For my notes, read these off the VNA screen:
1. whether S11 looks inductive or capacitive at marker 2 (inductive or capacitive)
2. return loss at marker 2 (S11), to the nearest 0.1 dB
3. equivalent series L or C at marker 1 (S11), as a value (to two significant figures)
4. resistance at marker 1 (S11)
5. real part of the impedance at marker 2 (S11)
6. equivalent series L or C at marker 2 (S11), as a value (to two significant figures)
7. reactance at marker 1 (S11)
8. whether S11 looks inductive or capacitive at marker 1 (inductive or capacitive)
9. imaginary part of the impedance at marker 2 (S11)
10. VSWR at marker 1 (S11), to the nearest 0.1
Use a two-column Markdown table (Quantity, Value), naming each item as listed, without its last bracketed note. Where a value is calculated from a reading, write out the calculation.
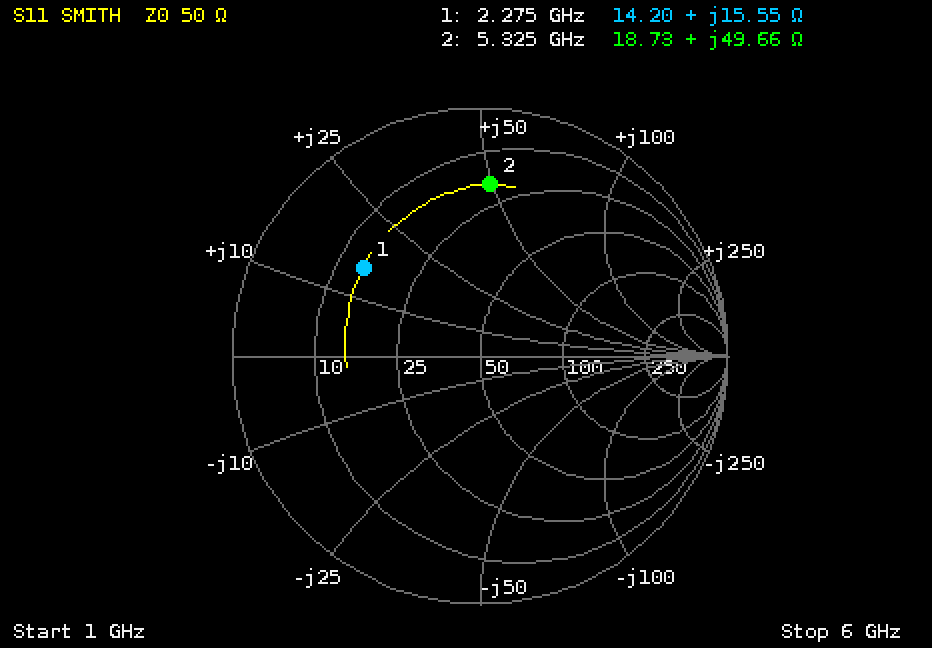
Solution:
| Quantity | Value |
|---|---|
| whether S11 looks inductive or capacitive at marker 2 | inductive |
| return loss at marker 2 (S11), to the nearest 0.1 dB | 3.2 dB |
| equivalent series L or C at marker 1 (S11), as a value | L = 15.55 Ω/(2π × 2.275 GHz) ≈ 1.1 nH |
| resistance at marker 1 | 14.20 Ω |
| real part of the impedance at marker 2 | 18.73 Ω |
| equivalent series L or C at marker 2 (S11), as a value | L = 49.66 Ω/(2π × 5.325 GHz) ≈ 1.5 nH |
| reactance at marker 1 | +15.55 Ω |
| whether S11 looks inductive or capacitive at marker 1 | inductive |
| imaginary part of the impedance at marker 2 | +49.66 Ω |
| VSWR at marker 1 (S11), to the nearest 0.1 | 3.9 |
